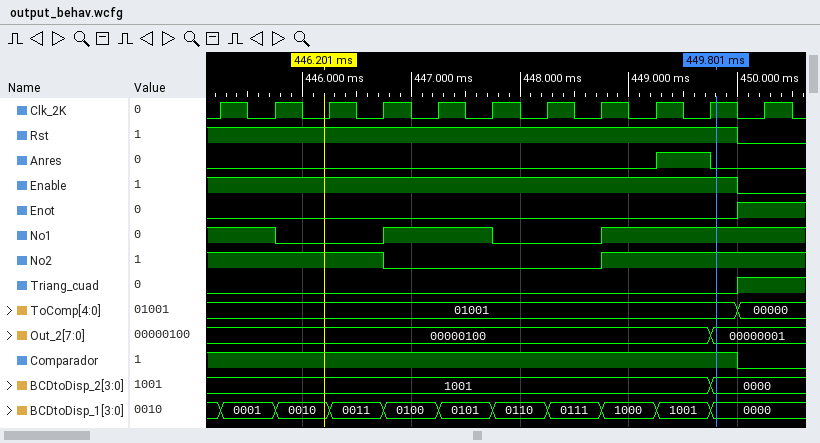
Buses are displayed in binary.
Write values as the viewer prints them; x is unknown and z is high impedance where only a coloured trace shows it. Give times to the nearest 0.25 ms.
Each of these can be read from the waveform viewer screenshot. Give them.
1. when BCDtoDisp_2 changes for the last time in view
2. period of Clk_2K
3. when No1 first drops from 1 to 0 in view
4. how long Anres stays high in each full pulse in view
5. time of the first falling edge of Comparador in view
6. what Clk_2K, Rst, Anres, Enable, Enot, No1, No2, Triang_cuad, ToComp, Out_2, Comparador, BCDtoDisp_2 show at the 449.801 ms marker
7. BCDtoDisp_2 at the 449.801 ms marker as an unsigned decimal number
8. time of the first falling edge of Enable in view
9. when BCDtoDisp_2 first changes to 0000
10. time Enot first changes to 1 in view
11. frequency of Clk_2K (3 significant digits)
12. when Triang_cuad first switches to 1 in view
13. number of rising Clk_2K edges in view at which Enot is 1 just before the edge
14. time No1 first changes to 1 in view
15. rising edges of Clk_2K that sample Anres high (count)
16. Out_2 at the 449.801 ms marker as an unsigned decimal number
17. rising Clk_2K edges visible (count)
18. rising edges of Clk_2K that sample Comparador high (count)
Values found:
449.75 ms
0.5 ms
445.75 ms
0.5 ms
450 ms
Clk_2K=1, Rst=1, Anres=0, Enable=1, Enot=0, No1=1, No2=1, Triang_cuad=0, ToComp=01001, Out_2=00000001, Comparador=1, BCDtoDisp_2=0000
0
450 ms
449.75 ms
450 ms
2.00 kHz
450 ms
1
446.75 ms
1
1
11
10
